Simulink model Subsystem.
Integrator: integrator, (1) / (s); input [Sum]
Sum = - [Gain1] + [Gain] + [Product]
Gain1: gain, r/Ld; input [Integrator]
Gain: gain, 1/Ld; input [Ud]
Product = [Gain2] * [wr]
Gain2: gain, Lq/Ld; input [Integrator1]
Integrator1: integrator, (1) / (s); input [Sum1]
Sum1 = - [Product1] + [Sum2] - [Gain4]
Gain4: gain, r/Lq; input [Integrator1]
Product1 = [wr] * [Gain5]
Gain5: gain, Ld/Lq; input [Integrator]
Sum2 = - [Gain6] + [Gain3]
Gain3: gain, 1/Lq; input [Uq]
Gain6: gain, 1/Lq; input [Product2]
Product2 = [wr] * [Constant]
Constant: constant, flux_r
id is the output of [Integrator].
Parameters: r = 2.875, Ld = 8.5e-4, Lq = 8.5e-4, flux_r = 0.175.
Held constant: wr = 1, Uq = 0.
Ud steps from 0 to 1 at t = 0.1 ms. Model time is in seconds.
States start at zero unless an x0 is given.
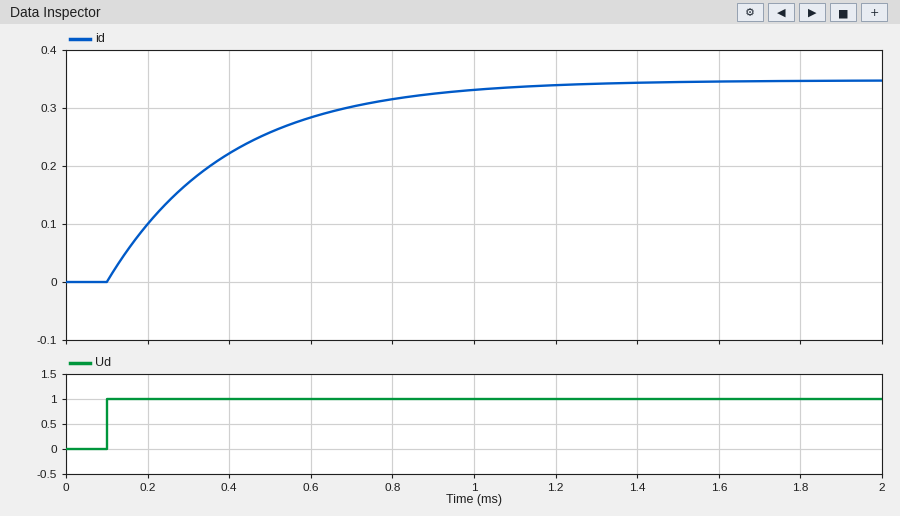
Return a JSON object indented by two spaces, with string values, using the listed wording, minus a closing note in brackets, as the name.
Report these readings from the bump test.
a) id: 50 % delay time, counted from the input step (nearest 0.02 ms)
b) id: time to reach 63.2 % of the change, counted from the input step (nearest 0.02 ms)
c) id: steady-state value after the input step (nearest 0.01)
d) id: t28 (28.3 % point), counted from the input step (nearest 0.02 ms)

{
  "id: 50 % delay time, counted from the input step": "0.20 ms",
  "id: time to reach 63.2 % of the change, counted from the input step": "0.30 ms",
  "id: steady-state value after the input step": "0.35",
  "id: t28 (28.3 % point), counted from the input step": "0.10 ms"
}
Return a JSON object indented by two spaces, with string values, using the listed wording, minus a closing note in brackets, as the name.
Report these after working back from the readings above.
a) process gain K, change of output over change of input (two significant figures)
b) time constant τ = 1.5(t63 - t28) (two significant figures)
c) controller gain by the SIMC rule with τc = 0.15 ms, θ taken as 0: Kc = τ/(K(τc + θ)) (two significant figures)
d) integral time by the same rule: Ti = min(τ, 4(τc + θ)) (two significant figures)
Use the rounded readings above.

{
  "process gain K, change of output over change of input": "0.35",
  "time constant τ = 1.5(t63 - t28)": "0.30 ms",
  "controller gain by the SIMC rule with τc = 0.15 ms, θ taken as 0: Kc = τ/(K(τc + θ))": "5.7",
  "integral time by the same rule: Ti = min(τ, 4(τc + θ))": "0.30 ms"
}
